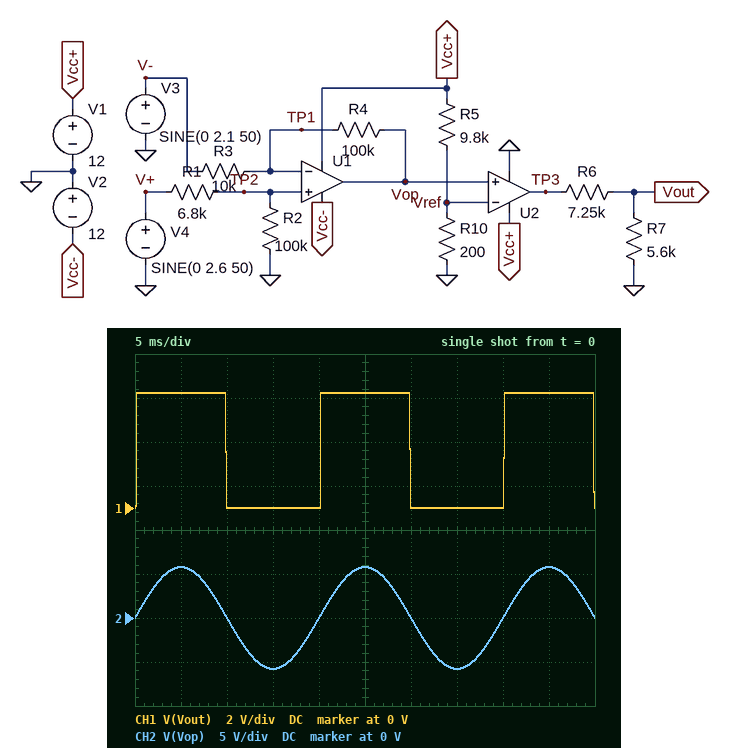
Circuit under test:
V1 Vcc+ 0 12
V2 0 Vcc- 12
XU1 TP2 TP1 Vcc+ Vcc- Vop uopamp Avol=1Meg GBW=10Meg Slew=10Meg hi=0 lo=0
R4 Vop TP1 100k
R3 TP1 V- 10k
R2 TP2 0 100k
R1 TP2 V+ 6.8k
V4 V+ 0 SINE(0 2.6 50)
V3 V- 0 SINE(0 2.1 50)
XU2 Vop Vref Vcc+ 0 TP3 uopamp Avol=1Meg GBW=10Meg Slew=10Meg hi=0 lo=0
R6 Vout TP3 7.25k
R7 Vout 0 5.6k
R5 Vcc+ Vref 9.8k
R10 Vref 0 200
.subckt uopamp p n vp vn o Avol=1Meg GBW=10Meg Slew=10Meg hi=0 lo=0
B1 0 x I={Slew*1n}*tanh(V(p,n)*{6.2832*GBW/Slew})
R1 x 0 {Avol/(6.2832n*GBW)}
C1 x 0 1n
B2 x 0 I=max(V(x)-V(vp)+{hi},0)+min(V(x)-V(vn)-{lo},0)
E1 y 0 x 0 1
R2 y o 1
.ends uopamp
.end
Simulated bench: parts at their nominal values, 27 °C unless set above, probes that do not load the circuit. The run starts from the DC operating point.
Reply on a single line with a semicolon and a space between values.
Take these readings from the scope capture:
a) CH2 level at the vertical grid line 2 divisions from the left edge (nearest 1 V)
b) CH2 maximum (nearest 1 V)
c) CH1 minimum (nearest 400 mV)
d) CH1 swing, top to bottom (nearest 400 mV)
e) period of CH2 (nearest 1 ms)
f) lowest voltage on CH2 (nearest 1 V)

0 V; 6 V; 0 V; 5.2 V; 20 ms; -6 V
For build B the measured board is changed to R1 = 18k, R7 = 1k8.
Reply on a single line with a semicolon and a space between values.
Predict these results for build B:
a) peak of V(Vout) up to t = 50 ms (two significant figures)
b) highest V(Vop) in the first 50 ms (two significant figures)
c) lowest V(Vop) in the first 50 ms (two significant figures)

2.4 V; 3.2 V; -3.2 V
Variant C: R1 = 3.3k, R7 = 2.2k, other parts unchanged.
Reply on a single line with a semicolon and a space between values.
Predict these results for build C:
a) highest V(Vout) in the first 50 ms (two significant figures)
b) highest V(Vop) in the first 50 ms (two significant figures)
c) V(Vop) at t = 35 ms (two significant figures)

2.8 V; 6.7 V; -6.7 V
